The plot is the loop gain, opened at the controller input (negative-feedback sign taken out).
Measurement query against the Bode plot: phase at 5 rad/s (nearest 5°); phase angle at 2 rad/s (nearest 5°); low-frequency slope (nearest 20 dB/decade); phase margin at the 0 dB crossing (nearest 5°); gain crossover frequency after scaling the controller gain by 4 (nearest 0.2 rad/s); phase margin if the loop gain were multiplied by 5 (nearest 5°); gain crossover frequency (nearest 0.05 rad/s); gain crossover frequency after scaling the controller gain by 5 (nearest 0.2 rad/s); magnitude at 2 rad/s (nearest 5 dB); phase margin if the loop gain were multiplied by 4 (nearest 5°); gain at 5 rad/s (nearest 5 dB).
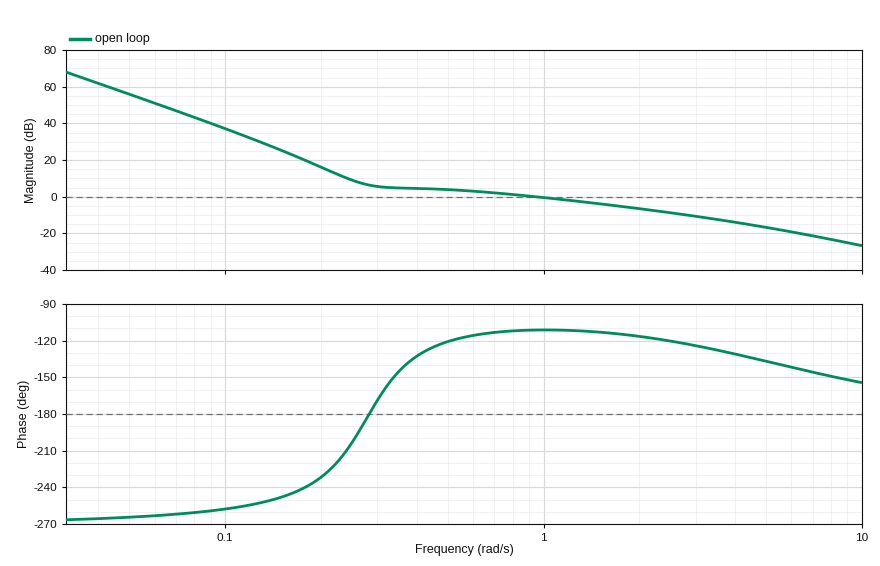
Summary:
-135°
-115°
-60 dB/decade
70°
3.4 rad/s
50°
0.95 rad/s
4.0 rad/s
-5 dB
55°
-15 dB
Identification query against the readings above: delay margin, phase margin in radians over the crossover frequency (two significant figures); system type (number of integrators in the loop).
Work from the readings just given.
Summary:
1.3 s
3
